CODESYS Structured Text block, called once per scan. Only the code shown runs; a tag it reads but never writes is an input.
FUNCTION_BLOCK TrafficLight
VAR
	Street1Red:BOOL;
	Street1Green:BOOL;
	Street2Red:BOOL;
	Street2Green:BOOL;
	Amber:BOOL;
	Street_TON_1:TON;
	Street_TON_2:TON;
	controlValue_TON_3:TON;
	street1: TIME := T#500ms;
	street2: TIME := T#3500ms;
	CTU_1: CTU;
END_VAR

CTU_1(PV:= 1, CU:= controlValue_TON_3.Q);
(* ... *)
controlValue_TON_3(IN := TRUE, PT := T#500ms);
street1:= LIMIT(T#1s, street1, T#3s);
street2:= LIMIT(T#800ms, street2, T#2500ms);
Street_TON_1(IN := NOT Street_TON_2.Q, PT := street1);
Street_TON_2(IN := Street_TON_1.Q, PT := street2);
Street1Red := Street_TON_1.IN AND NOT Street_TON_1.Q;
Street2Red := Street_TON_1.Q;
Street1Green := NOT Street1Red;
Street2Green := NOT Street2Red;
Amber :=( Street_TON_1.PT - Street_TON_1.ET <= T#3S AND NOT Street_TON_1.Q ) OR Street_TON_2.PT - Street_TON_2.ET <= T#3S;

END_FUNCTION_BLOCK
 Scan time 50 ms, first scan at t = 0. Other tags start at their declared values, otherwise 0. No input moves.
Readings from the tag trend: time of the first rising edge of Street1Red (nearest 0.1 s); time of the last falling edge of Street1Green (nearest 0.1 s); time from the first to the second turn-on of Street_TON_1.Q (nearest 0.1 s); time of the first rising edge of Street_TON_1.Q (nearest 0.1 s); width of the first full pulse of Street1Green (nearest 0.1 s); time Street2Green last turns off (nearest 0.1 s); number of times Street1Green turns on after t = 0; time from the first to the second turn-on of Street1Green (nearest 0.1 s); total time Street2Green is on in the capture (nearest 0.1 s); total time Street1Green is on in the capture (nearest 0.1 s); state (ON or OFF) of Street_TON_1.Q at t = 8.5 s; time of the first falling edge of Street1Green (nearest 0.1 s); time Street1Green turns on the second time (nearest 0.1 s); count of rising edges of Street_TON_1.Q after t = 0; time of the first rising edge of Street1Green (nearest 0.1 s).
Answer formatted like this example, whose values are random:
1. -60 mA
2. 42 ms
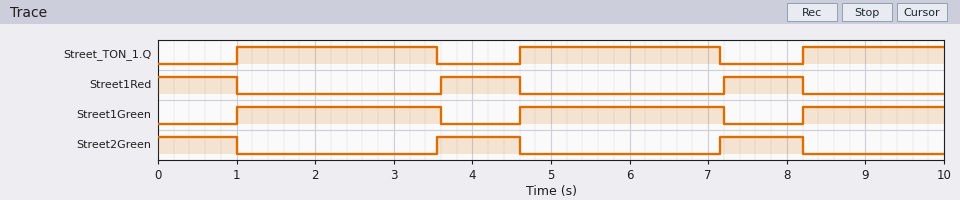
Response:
1. 3.6 s
2. 7.2 s
3. 3.6 s
4. 1.0 s
5. 2.6 s
6. 8.2 s
7. 3
8. 3.6 s
9. 3.1 s
10. 7.0 s
11. ON
12. 3.6 s
13. 4.6 s
14. 3
15. 1.0 s
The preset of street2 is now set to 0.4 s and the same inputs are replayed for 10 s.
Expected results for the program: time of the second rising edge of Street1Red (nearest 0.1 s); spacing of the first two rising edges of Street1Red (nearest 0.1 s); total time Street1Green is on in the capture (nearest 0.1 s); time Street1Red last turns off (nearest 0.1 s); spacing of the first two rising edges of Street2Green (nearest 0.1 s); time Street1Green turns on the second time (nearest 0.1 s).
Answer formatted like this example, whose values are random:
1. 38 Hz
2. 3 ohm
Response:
1. 3.8 s
2. 1.9 s
3. 4.5 s
4. 8.6 s
5. 1.9 s
6. 2.9 s
